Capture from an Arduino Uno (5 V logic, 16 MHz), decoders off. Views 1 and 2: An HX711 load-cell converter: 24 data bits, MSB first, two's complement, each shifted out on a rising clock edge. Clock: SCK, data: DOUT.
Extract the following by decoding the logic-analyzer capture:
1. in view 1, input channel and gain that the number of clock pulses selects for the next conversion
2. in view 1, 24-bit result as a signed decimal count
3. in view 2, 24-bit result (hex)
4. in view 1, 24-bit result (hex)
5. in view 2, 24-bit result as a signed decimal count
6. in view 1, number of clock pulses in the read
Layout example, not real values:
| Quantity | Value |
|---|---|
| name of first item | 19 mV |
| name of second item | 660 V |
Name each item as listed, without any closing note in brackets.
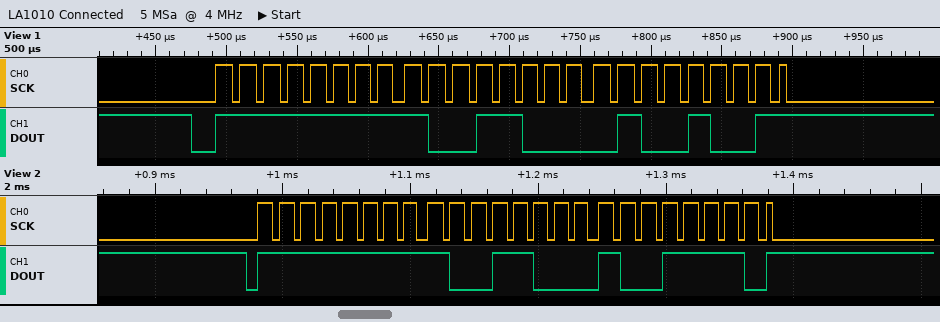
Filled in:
| Quantity | Value |
|---|---|
| in view 1, input channel and gain that the number of clock pulses selects for the next conversion | channel A, gain 128 |
| in view 1, 24-bit result as a signed decimal count | -26551 |
| in view 2, 24-bit result | 0xFF989E |
| in view 1, 24-bit result | 0xFF9849 |
| in view 2, 24-bit result as a signed decimal count | -26466 |
| in view 1, number of clock pulses in the read | 25 |
